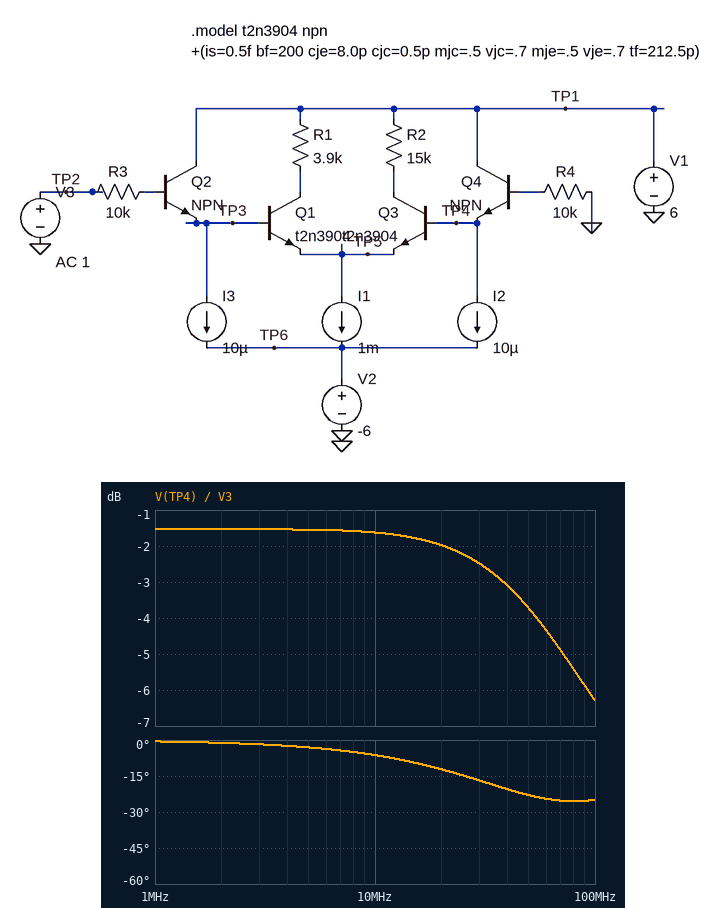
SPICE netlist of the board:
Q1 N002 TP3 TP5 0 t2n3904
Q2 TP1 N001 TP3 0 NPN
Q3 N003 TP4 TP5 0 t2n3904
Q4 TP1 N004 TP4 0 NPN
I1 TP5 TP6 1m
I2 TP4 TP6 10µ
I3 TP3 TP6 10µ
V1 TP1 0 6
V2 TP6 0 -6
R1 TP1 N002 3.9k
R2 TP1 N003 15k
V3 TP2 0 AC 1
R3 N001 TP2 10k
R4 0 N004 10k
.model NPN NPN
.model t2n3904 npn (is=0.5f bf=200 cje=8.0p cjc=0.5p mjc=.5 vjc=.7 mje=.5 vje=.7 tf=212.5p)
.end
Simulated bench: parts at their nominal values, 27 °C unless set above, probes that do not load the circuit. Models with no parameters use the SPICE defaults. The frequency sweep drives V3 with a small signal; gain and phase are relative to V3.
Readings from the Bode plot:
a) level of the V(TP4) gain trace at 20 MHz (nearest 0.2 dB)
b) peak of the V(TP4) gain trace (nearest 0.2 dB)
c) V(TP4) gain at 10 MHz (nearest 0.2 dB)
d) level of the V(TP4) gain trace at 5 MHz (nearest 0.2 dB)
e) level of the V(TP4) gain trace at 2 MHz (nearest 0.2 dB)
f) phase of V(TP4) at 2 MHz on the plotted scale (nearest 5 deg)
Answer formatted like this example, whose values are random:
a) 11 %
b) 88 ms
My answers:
a) -2.0 dB
b) -1.6 dB
c) -1.6 dB
d) -1.6 dB
e) -1.6 dB
f) 0 deg
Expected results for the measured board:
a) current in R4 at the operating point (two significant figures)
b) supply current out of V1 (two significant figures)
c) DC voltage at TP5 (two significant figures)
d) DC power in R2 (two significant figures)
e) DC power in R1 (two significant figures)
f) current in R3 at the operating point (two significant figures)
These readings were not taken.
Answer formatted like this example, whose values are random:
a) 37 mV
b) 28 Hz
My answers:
a) 130 nA
b) 1.0 mA
c) -1.4 V
d) 3.5 mW
e) 1.0 mW
f) 120 nA
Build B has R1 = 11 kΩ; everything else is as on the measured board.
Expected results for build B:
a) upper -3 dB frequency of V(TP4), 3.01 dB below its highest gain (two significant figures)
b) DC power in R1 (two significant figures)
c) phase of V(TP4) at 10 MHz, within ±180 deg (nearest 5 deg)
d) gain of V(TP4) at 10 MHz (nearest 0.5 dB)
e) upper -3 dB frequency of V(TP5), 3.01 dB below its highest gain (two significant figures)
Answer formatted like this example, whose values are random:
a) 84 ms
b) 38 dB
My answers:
a) 19 MHz
b) 2.9 mW
c) -15 deg
d) -3.5 dB
e) 14 MHz
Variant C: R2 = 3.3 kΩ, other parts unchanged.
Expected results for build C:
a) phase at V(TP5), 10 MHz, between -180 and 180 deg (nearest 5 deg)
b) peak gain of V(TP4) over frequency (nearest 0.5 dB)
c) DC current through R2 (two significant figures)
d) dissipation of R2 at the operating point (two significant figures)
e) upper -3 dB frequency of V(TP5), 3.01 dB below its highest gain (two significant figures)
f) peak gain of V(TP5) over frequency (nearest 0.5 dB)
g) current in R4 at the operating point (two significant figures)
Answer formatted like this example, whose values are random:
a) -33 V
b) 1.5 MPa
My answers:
a) 0 deg
b) -6.5 dB
c) 500 µA
d) 820 µW
e) 330 MHz
f) -6.0 dB
g) 120 nA
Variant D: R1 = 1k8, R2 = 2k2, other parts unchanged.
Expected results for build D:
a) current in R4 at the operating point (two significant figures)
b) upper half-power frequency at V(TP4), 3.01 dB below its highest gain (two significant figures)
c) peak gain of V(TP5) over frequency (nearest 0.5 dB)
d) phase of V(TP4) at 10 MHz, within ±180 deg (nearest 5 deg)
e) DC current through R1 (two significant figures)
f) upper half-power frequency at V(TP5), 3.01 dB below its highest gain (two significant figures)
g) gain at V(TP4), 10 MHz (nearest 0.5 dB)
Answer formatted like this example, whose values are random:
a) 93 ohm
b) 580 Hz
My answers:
a) 120 nA
b) 310 MHz
c) -6.0 dB
d) 15 deg
e) 500 µA
f) 300 MHz
g) -6.5 dB
